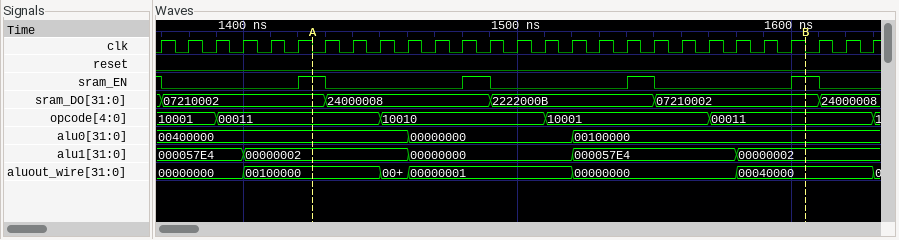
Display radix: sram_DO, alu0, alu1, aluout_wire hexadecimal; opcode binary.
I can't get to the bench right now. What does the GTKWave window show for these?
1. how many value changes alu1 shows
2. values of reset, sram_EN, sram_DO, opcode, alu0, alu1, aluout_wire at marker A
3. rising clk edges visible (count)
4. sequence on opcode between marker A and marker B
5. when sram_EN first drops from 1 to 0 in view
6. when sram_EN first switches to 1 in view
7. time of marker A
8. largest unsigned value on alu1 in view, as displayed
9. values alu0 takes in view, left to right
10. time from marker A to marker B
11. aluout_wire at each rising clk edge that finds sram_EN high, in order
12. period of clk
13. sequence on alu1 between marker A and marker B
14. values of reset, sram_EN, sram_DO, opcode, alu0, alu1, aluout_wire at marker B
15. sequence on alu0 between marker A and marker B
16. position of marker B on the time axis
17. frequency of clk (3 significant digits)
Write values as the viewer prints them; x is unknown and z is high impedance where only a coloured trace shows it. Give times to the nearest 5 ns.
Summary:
4
reset=0, sram_EN=1, sram_DO=07210002, opcode=00011, alu0=00400000, alu1=00000002, aluout_wire=00100000
27
00011, 10010, 10001, 00011
1370 ns
1420 ns
1425 ns
000057E4
00400000, 00000000, 00100000
180 ns
00000000, 00100000, 00000001, 00000000, 00040000
10 ns
00000002, 00000000, 000057E4, 00000002
reset=0, sram_EN=1, sram_DO=07210002, opcode=00011, alu0=00100000, alu1=00000002, aluout_wire=00040000
00400000, 00000000, 00100000
1605 ns
100 MHz
